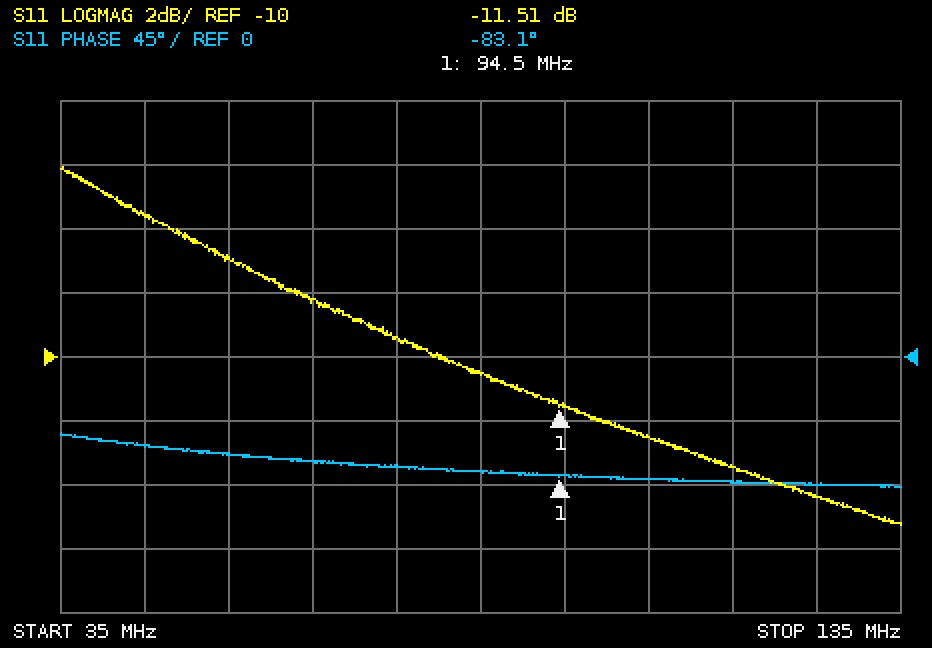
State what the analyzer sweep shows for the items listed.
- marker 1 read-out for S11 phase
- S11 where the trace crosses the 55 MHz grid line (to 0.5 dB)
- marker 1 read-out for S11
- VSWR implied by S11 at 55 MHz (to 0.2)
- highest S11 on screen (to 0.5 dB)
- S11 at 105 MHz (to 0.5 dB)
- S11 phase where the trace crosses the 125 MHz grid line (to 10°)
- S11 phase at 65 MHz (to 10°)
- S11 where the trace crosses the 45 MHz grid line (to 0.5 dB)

-83.1°
-7.0 dB
-11.51 dB
2.6
-4.0 dB
-12.5 dB
-90°
-70°
-5.5 dB
